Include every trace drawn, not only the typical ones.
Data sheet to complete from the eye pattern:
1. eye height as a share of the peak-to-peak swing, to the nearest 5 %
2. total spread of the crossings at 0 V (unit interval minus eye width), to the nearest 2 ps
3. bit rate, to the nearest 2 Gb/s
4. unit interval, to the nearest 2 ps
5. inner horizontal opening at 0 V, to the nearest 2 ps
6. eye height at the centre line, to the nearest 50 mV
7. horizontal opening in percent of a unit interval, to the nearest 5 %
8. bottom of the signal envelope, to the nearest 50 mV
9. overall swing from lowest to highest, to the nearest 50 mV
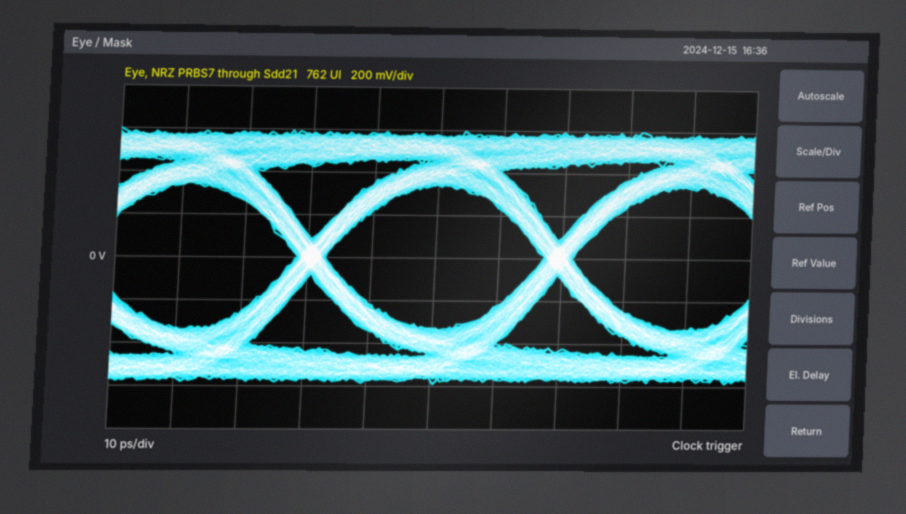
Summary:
55 %
4 ps
26 Gb/s
38 ps
34 ps
650 mV
90 %
-600 mV
1.20 V
